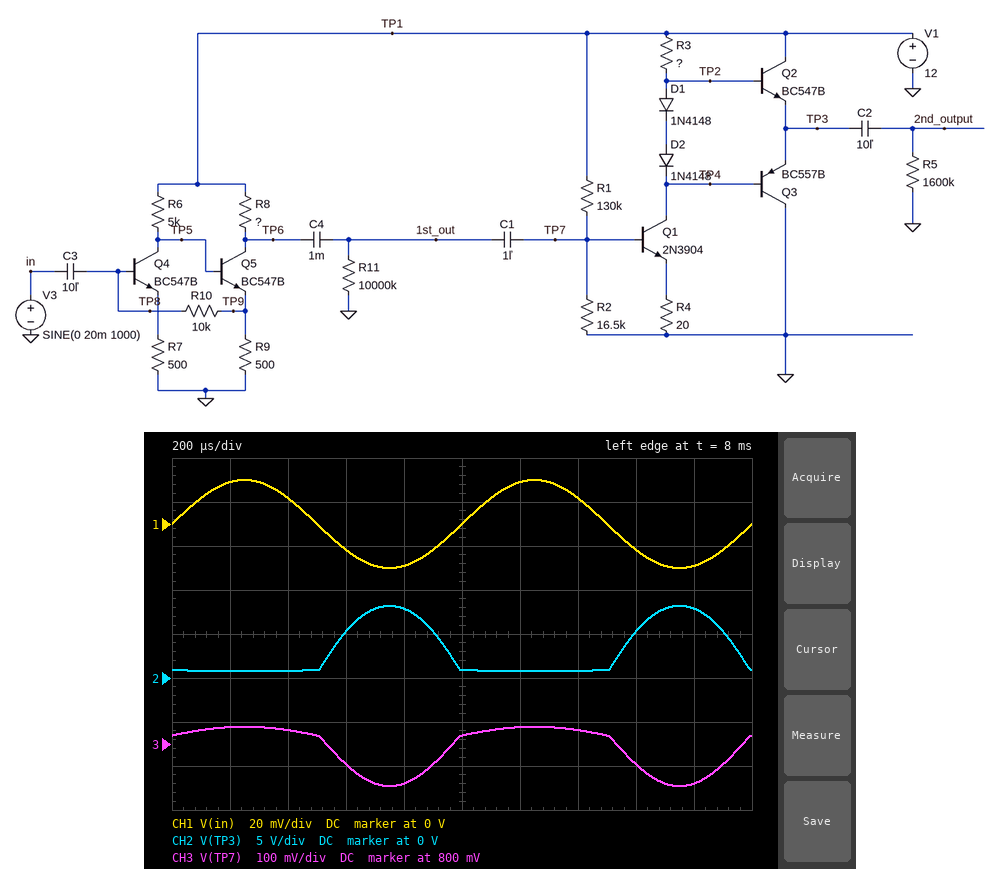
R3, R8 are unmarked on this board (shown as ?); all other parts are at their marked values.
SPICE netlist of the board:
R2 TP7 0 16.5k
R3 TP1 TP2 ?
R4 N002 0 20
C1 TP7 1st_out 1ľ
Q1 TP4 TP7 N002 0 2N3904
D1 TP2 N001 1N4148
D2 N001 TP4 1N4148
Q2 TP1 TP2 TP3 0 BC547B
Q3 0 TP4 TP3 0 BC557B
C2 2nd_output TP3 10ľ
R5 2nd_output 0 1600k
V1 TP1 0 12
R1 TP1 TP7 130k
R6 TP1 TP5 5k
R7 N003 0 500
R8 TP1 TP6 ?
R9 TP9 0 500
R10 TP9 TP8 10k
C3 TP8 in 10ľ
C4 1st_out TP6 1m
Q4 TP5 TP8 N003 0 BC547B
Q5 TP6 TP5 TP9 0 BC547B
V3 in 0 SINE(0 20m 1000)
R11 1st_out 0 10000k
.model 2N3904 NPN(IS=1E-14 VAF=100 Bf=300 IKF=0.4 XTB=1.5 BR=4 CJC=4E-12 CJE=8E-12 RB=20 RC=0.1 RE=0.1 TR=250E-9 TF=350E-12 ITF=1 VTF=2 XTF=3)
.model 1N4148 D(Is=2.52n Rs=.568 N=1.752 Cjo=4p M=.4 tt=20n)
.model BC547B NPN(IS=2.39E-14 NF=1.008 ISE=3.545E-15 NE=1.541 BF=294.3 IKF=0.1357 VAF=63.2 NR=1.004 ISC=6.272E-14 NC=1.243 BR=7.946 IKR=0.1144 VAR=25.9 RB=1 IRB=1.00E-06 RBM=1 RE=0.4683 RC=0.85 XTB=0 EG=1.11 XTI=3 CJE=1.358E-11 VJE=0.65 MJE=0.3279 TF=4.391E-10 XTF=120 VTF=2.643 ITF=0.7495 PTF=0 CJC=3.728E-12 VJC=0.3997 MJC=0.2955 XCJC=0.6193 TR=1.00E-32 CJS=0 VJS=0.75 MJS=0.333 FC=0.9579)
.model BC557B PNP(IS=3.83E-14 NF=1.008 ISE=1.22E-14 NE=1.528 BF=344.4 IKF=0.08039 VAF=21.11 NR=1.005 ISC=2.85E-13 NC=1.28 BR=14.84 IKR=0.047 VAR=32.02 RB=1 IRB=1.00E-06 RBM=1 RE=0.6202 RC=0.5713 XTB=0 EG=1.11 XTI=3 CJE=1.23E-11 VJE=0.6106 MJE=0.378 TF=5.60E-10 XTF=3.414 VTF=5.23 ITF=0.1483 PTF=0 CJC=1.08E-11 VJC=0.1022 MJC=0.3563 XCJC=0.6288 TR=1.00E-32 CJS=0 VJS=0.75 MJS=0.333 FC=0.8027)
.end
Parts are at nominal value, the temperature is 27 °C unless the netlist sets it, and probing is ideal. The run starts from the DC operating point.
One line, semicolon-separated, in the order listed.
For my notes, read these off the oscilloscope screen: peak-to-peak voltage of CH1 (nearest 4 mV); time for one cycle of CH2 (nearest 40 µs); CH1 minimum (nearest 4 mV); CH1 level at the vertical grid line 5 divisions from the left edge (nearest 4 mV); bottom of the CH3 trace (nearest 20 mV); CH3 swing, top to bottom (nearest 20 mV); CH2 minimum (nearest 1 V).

40 mV; 1.00 ms; -20 mV; 0 V; 700 mV; 140 mV; 1 V
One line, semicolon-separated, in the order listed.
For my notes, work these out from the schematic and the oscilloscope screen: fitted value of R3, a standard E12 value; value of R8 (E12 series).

1.8 kΩ; 330 Ω
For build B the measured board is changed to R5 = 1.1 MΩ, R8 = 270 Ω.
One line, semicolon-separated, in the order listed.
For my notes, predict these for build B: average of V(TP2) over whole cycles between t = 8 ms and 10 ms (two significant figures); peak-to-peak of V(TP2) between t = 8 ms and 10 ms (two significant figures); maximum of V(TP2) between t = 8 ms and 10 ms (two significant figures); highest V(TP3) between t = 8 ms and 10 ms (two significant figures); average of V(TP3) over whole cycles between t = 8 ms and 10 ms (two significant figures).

3.5 V; 6.2 V; 7.7 V; 7.1 V; 2.8 V
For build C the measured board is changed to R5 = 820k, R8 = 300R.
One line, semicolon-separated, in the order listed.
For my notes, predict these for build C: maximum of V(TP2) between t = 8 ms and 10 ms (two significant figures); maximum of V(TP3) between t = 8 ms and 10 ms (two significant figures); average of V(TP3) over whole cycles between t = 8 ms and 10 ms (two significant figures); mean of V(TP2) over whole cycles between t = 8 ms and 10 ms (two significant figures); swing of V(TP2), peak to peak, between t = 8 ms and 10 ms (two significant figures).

8.3 V; 7.7 V; 3.0 V; 3.7 V; 6.8 V
